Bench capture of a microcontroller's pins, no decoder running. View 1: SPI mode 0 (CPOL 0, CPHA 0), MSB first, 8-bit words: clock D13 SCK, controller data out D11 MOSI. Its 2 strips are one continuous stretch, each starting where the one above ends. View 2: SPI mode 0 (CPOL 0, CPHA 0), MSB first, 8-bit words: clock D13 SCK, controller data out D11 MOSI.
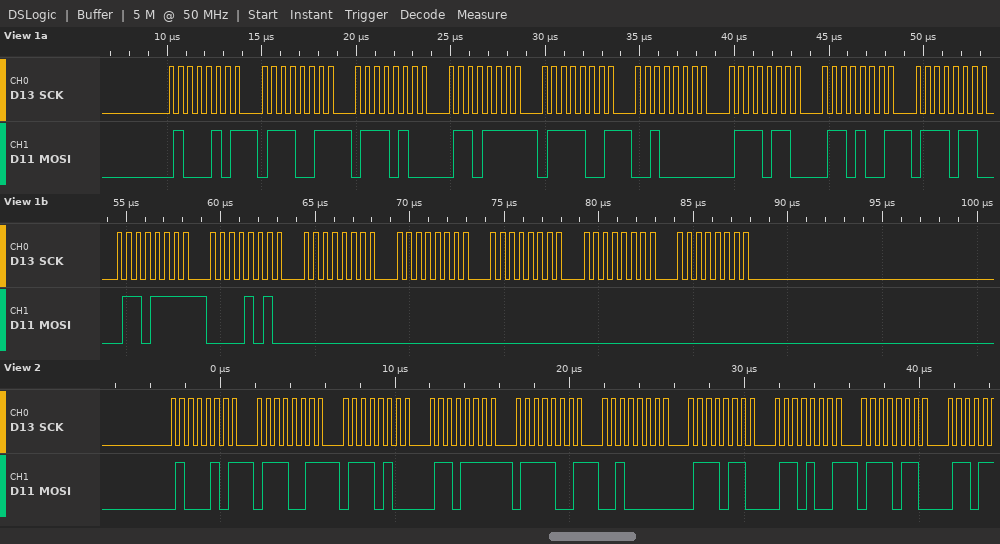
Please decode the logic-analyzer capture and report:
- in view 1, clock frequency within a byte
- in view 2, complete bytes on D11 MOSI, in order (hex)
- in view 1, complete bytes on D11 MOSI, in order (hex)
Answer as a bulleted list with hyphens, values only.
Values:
- 2 MHz
- 0x45 0x73 0x74 0x6F 0x79 0x20 0x76 0x69 0x76
- 45 73 74 6F 79 20 76 69 76 6F 0A 00 00 00 00 00
